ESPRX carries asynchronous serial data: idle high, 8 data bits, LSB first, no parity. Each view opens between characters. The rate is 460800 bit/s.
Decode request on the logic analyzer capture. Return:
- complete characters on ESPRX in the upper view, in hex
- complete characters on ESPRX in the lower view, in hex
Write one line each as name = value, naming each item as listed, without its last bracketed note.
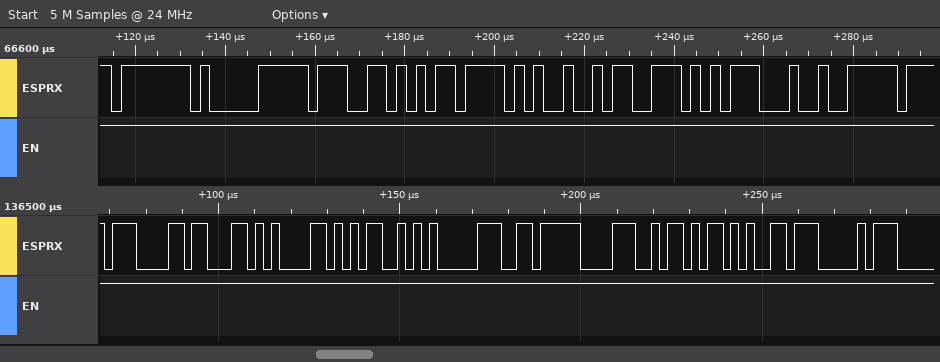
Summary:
complete characters on ESPRX in the upper view, in hex = 7F, F0, 67, ED, 25, 73, 1D, F2
complete characters on ESPRX in the lower view, in hex = 87, 63, 61, 4D, C1, F6, 38, 6B, D9, D0
